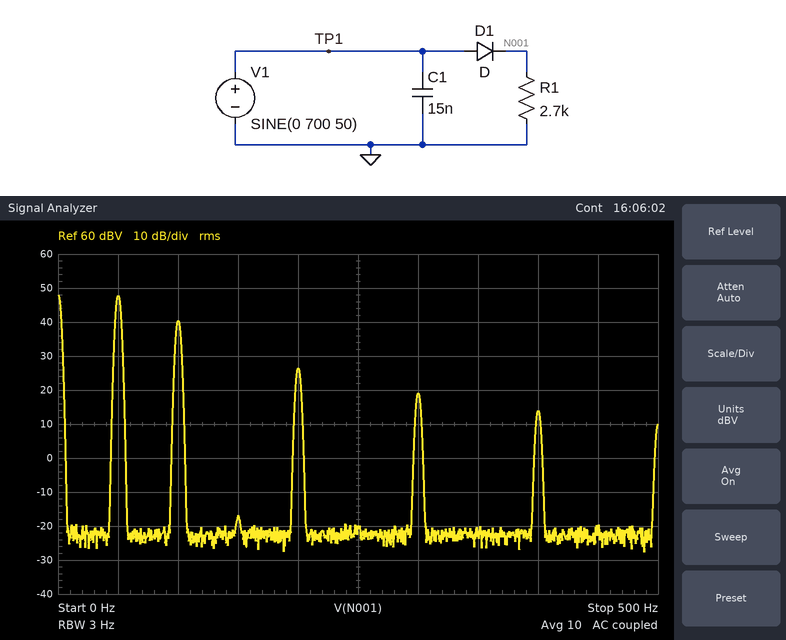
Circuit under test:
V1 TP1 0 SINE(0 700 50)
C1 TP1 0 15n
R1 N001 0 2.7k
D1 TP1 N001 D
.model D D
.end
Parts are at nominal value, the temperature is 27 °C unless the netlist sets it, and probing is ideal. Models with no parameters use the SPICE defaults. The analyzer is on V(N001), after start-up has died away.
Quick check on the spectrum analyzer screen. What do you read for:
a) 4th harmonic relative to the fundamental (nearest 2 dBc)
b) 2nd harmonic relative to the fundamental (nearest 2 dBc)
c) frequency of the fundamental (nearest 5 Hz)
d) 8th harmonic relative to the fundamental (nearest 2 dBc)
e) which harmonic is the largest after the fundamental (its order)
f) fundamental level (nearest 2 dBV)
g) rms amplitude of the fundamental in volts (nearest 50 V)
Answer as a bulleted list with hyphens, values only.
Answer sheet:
- -22 dBc
- -8 dBc
- 50 Hz
- -34 dBc
- 2
- 48 dBV
- 250 V
